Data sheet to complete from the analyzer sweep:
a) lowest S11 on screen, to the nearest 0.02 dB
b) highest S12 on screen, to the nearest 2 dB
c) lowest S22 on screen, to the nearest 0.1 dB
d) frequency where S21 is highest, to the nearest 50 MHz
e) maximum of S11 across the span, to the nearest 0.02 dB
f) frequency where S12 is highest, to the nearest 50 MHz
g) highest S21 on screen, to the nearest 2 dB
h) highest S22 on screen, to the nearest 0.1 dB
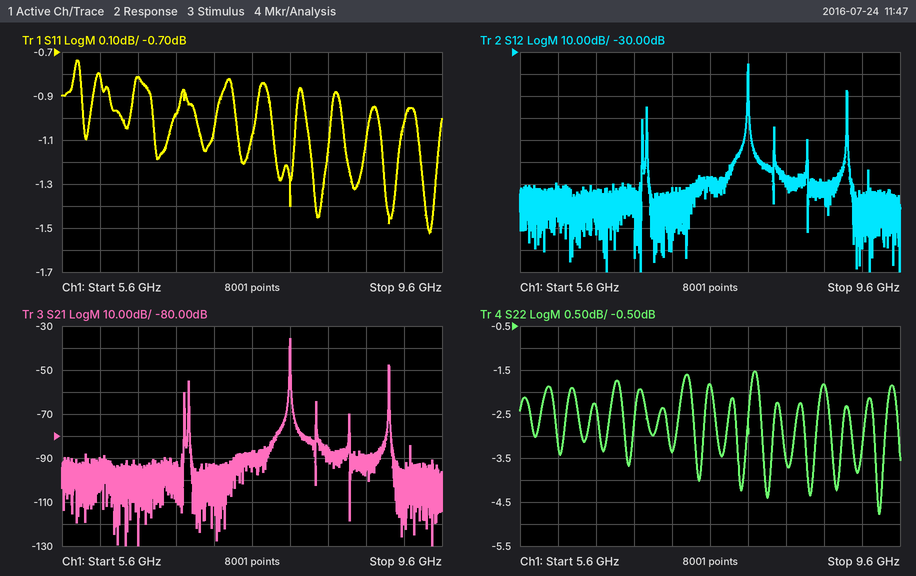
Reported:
-1.52 dB
-36 dB
-4.8 dB
8.00 GHz
-0.74 dB
8.00 GHz
-36 dB
-1.5 dB
